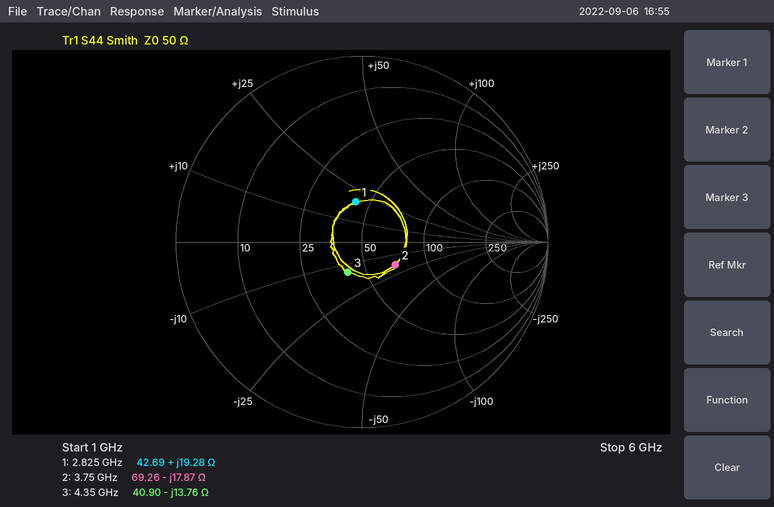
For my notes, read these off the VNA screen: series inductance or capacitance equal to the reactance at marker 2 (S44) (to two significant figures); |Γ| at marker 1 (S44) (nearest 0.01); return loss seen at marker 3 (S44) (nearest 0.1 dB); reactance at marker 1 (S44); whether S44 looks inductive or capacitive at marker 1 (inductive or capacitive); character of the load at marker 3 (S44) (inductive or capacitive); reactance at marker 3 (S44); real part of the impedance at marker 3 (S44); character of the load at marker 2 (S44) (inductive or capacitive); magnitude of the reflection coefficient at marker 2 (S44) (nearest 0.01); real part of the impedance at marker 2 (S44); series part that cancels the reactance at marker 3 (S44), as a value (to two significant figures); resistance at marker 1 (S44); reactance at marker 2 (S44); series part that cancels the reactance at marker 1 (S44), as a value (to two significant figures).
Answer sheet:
2.4 pF
0.22
14.9 dB
+19.28 Ω
inductive
capacitive
-13.76 Ω
40.90 Ω
capacitive
0.22
69.26 Ω
500 pH
42.69 Ω
-17.87 Ω
2.9 pF
